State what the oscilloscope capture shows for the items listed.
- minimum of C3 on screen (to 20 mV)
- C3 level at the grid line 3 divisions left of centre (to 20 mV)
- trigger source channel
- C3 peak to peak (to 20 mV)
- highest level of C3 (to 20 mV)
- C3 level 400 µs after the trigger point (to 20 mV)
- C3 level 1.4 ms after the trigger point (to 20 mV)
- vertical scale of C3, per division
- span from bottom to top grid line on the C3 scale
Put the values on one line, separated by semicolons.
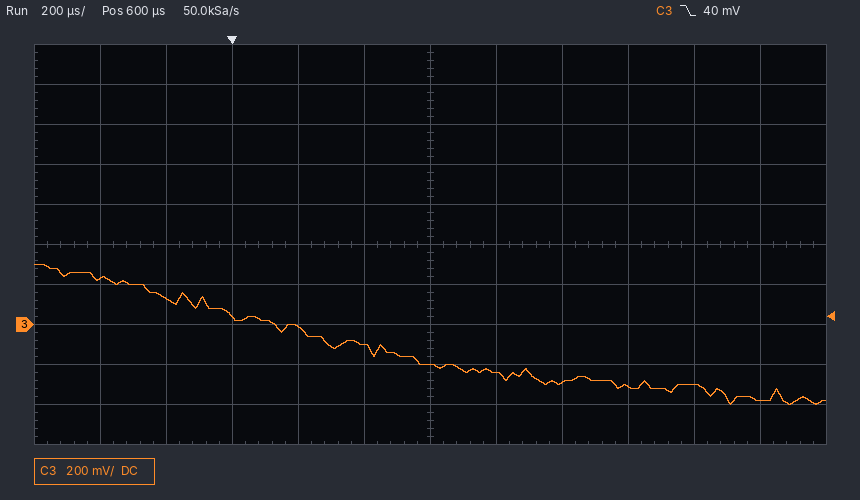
-400 mV; 40 mV; C3; 700 mV; 300 mV; -100 mV; -300 mV; 200 mV; 2 V
